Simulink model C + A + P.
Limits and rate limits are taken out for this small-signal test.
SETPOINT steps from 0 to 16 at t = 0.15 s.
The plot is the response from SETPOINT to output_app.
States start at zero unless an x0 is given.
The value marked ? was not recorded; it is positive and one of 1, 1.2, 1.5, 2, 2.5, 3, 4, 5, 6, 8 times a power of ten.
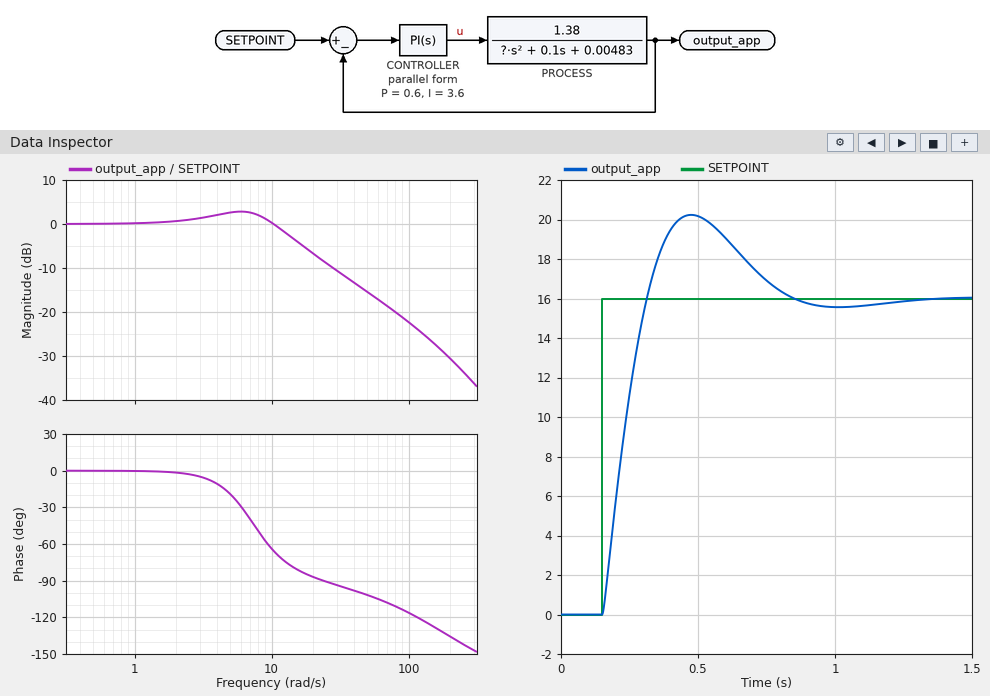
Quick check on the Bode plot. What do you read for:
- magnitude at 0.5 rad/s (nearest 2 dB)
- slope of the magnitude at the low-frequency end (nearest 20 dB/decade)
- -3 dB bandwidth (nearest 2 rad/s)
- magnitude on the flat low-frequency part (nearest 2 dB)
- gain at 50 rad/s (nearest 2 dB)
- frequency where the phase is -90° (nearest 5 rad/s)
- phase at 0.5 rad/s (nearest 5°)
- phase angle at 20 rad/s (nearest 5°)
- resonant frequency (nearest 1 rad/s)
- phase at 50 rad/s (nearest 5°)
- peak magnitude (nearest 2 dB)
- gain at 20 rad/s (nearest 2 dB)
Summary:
0 dB
0 dB/decade
14 rad/s
0 dB
-16 dB
25 rad/s
0°
-85°
6 rad/s
-100°
2 dB
-6 dB
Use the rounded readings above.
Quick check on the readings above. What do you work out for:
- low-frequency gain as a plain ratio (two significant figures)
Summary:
1.0
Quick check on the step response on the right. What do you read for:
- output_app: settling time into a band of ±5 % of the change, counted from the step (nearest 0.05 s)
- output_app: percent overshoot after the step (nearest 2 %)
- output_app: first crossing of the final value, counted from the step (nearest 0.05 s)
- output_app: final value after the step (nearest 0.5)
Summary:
0.60 s
26 %
0.15 s
16.0
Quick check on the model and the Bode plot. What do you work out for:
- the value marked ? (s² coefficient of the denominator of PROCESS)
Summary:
0.0005
